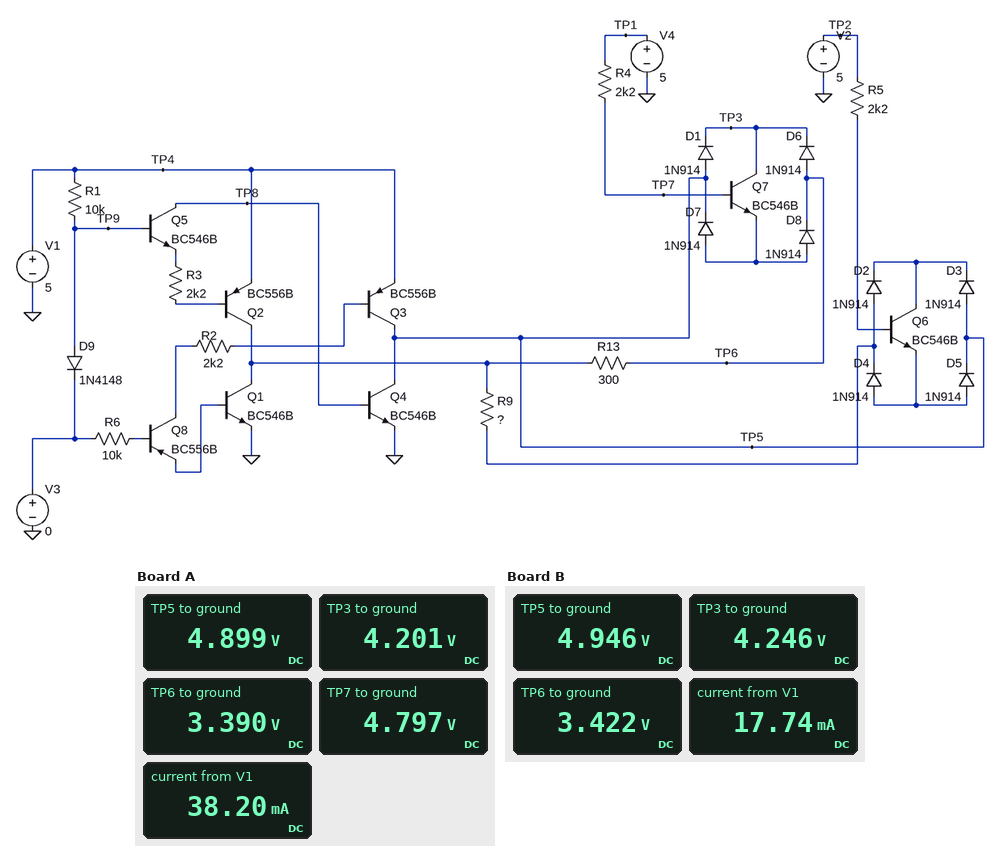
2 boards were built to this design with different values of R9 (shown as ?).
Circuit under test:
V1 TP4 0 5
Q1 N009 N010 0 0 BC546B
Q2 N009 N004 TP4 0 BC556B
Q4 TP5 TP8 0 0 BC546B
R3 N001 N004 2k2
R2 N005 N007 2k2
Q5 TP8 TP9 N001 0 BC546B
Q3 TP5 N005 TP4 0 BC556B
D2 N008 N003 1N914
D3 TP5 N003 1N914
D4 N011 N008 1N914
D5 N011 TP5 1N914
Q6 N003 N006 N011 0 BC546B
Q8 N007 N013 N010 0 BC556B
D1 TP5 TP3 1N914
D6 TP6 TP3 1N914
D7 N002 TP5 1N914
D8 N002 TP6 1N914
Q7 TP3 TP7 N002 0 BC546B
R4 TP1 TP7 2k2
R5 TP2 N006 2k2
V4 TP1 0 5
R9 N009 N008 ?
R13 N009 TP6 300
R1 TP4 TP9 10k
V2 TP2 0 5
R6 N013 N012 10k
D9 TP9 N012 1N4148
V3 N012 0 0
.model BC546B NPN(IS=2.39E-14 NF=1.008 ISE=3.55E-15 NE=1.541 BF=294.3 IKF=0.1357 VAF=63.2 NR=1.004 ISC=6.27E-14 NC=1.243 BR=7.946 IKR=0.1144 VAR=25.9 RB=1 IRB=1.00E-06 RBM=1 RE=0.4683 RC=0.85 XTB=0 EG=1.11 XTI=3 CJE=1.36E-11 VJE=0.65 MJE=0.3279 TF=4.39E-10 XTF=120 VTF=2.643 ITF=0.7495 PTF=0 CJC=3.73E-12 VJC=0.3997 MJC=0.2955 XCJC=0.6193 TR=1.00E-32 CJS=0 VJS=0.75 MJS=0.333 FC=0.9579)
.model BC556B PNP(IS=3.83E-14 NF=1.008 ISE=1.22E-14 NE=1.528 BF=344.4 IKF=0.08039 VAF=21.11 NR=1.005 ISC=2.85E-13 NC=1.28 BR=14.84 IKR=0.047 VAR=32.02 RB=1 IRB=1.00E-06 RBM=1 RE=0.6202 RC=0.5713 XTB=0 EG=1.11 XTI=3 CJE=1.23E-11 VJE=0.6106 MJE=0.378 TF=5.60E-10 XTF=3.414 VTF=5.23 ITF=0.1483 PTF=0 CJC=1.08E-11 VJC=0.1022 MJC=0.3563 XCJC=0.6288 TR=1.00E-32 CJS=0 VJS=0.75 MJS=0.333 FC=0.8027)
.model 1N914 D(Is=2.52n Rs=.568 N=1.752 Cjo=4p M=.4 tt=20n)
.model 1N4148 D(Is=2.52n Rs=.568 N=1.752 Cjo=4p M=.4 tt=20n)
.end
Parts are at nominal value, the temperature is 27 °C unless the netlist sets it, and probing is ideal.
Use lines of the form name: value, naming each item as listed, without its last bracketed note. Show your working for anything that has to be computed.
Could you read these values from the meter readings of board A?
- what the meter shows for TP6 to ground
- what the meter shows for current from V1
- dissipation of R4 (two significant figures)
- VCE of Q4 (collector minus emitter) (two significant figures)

what the meter shows for TP6 to ground: 3.390 V
what the meter shows for current from V1: 38.20 mA
dissipation of R4: (5 V - 4.797 V)^2 / 2.2 kΩ = 19 µW
VCE of Q4 (collector minus emitter): 4.899 V = 4.9 V
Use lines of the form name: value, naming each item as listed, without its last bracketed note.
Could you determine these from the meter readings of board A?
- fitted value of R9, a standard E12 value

fitted value of R9, a standard E12 value: 120 Ω
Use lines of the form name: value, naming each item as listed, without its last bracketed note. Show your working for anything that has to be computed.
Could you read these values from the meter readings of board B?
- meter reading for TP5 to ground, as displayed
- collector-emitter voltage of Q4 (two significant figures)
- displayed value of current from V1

meter reading for TP5 to ground, as displayed: 4.946 V
collector-emitter voltage of Q4: 4.946 V = 4.9 V
displayed value of current from V1: 17.74 mA
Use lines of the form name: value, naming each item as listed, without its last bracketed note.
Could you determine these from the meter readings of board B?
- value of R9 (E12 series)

value of R9: 680 Ω
